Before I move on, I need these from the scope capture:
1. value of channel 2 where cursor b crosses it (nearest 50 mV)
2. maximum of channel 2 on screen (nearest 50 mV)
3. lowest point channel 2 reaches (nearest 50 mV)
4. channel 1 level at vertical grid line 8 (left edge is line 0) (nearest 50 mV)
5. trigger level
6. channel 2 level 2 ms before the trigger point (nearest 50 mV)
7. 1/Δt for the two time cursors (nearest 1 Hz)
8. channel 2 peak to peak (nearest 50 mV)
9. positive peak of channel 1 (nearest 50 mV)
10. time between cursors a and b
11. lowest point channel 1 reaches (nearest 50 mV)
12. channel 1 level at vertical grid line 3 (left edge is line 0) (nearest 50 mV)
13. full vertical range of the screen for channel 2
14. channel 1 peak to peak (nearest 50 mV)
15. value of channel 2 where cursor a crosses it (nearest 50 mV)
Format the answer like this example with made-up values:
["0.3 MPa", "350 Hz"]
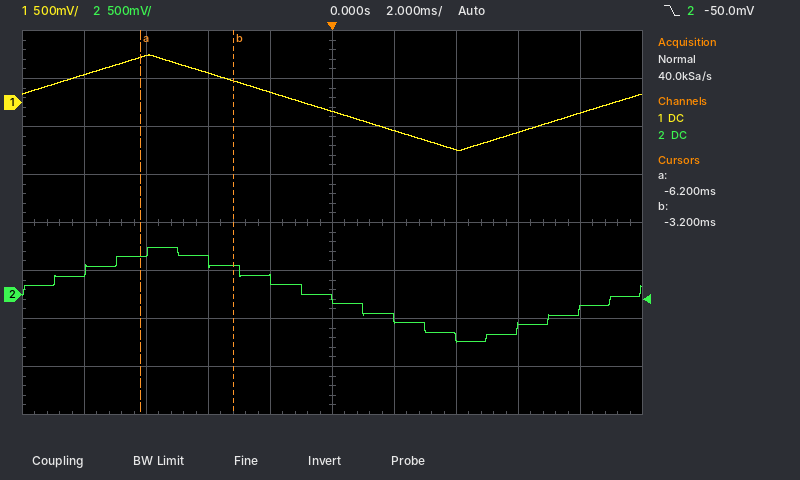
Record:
["300 mV", "500 mV", "-500 mV", "-300 mV", "-50.0 mV", "150 mV", "333 Hz", "1.00 V", "500 mV", "3.0 ms", "-500 mV", "300 mV", "4 V", "1.00 V", "400 mV"]
